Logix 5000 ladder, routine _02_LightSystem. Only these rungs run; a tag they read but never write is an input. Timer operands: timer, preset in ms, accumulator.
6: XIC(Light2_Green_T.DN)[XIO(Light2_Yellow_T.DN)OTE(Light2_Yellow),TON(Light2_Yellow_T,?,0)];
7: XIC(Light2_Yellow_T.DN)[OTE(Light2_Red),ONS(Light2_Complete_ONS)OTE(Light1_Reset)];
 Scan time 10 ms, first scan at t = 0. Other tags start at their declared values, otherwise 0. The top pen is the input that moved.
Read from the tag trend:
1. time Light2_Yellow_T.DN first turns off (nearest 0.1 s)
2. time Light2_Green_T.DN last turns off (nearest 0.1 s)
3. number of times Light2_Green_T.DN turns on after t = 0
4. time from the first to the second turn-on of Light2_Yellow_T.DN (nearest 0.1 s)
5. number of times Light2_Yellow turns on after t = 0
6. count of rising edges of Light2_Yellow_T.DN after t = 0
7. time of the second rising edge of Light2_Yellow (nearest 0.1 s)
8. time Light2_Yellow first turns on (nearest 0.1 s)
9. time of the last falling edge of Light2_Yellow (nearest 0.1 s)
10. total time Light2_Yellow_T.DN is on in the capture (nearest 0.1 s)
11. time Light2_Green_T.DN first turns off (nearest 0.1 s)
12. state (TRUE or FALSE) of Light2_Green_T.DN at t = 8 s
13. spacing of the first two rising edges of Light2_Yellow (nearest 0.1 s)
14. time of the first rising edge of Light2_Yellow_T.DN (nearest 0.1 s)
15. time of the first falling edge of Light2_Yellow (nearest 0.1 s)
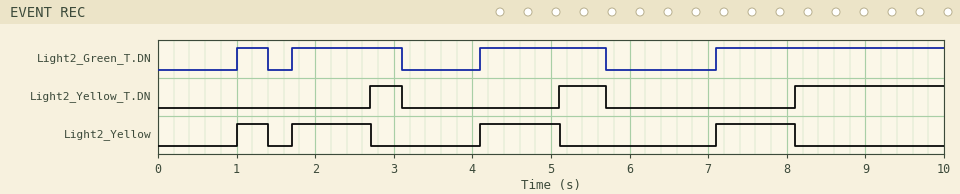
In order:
3.1 s
5.7 s
4
2.4 s
4
3
1.7 s
1.0 s
8.1 s
2.9 s
1.4 s
TRUE
0.7 s
2.7 s
1.4 s
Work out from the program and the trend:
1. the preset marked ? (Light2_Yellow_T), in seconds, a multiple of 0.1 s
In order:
1.0 s
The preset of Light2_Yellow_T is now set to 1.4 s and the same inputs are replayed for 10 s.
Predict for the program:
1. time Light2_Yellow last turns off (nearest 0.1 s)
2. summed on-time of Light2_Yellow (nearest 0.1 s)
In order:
8.5 s
4.6 s
